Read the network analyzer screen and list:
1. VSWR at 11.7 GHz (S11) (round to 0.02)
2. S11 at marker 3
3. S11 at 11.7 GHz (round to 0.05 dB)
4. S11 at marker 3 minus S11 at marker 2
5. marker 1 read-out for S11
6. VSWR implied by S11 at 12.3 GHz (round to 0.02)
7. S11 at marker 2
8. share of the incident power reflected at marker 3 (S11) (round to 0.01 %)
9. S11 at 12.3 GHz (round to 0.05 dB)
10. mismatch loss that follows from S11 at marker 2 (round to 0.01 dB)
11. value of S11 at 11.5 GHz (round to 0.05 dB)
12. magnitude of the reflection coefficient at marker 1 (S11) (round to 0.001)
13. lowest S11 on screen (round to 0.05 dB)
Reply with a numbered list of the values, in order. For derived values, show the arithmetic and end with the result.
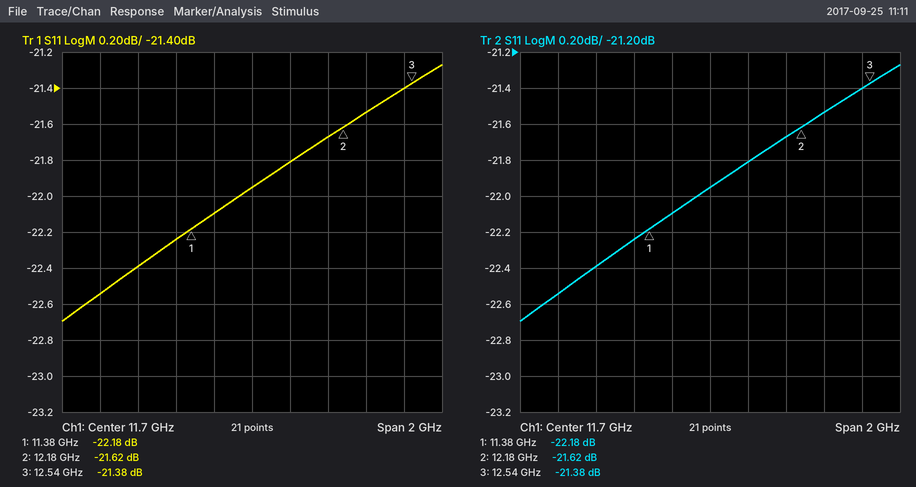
1. |Γ| = 10^(-21.95/20) = 0.0799; VSWR = (1 + 0.0799)/(1 − 0.0799) ≈ 1.17, so 1.18 to the nearest 0.02
2. -21.38 dB
3. -21.95 dB
4. -21.38 − (-21.62) = 0.24 dB
5. -22.18 dB
6. |Γ| = 10^(-21.55/20) = 0.0837; VSWR = (1 + 0.0837)/(1 − 0.0837) ≈ 1.18
7. -21.62 dB
8. 10^(-21.38/10) ≈ 0.73 %
9. -21.55 dB
10. −10 log10(1 − 10^(-21.62/10)) ≈ 0.03 dB
11. -22.10 dB
12. 10^(-22.18/20) ≈ 0.078
13. -22.70 dB
